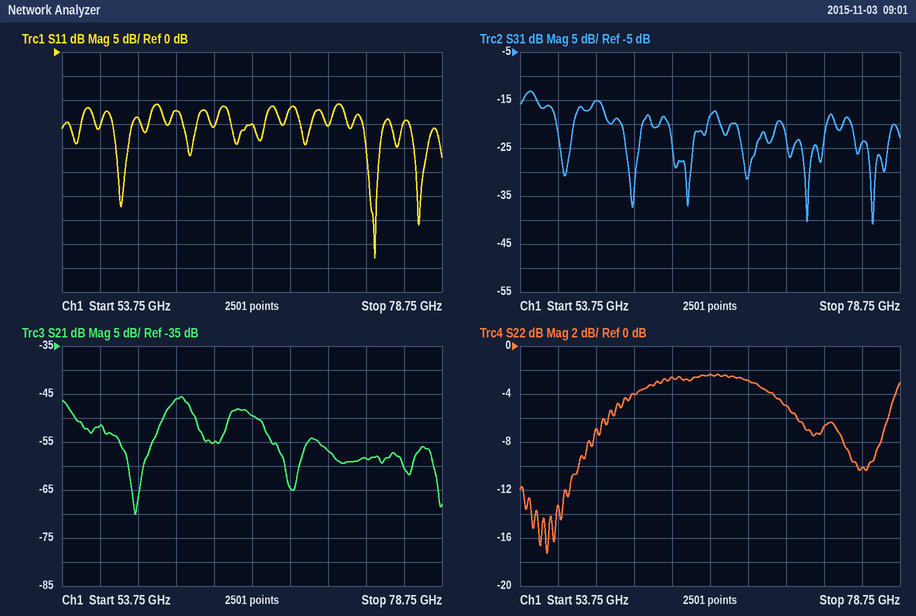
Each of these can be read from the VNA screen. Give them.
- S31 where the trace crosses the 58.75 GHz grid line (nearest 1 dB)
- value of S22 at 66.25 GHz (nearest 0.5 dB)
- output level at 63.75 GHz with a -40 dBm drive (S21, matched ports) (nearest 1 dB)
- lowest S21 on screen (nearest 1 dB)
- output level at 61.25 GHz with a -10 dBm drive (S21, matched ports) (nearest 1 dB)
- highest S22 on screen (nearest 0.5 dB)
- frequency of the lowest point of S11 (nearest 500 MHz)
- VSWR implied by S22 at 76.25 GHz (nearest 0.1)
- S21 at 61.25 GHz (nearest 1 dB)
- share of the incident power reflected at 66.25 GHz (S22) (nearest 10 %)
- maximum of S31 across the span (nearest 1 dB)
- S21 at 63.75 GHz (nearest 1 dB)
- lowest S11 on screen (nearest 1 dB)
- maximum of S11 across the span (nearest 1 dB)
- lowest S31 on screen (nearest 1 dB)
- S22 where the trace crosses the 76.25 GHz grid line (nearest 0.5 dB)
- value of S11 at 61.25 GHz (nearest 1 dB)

-15 dB
-2.5 dB
-95 dBm
-70 dB
-56 dBm
-2.5 dB
74.5 GHz
1.9
-46 dB
60 %
-13 dB
-55 dB
-43 dB
-11 dB
-41 dB
-10.0 dB
-12 dB
